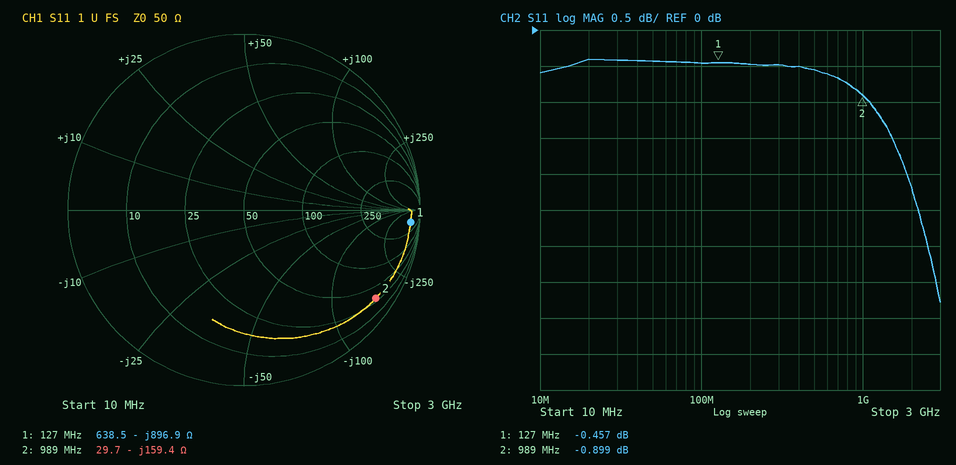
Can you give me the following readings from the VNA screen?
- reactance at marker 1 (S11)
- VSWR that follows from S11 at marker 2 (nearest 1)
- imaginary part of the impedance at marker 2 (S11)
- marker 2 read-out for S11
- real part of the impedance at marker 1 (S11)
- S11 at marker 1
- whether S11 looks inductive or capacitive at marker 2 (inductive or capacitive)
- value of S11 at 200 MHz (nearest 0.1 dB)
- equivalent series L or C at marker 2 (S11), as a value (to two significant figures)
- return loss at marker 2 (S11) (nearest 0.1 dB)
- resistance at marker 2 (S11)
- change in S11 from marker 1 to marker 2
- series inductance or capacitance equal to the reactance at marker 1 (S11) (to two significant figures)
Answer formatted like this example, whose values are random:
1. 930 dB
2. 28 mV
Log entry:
1. -896.9 Ω
2. 19
3. -159.4 Ω
4. -0.899 dB
5. 638.5 Ω
6. -0.457 dB
7. capacitive
8. -0.5 dB
9. 1.0 pF
10. 0.9 dB
11. 29.7 Ω
12. -0.442 dB
13. 1.4 pF
